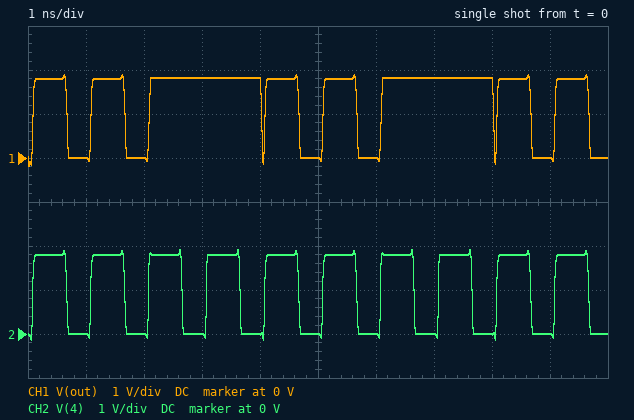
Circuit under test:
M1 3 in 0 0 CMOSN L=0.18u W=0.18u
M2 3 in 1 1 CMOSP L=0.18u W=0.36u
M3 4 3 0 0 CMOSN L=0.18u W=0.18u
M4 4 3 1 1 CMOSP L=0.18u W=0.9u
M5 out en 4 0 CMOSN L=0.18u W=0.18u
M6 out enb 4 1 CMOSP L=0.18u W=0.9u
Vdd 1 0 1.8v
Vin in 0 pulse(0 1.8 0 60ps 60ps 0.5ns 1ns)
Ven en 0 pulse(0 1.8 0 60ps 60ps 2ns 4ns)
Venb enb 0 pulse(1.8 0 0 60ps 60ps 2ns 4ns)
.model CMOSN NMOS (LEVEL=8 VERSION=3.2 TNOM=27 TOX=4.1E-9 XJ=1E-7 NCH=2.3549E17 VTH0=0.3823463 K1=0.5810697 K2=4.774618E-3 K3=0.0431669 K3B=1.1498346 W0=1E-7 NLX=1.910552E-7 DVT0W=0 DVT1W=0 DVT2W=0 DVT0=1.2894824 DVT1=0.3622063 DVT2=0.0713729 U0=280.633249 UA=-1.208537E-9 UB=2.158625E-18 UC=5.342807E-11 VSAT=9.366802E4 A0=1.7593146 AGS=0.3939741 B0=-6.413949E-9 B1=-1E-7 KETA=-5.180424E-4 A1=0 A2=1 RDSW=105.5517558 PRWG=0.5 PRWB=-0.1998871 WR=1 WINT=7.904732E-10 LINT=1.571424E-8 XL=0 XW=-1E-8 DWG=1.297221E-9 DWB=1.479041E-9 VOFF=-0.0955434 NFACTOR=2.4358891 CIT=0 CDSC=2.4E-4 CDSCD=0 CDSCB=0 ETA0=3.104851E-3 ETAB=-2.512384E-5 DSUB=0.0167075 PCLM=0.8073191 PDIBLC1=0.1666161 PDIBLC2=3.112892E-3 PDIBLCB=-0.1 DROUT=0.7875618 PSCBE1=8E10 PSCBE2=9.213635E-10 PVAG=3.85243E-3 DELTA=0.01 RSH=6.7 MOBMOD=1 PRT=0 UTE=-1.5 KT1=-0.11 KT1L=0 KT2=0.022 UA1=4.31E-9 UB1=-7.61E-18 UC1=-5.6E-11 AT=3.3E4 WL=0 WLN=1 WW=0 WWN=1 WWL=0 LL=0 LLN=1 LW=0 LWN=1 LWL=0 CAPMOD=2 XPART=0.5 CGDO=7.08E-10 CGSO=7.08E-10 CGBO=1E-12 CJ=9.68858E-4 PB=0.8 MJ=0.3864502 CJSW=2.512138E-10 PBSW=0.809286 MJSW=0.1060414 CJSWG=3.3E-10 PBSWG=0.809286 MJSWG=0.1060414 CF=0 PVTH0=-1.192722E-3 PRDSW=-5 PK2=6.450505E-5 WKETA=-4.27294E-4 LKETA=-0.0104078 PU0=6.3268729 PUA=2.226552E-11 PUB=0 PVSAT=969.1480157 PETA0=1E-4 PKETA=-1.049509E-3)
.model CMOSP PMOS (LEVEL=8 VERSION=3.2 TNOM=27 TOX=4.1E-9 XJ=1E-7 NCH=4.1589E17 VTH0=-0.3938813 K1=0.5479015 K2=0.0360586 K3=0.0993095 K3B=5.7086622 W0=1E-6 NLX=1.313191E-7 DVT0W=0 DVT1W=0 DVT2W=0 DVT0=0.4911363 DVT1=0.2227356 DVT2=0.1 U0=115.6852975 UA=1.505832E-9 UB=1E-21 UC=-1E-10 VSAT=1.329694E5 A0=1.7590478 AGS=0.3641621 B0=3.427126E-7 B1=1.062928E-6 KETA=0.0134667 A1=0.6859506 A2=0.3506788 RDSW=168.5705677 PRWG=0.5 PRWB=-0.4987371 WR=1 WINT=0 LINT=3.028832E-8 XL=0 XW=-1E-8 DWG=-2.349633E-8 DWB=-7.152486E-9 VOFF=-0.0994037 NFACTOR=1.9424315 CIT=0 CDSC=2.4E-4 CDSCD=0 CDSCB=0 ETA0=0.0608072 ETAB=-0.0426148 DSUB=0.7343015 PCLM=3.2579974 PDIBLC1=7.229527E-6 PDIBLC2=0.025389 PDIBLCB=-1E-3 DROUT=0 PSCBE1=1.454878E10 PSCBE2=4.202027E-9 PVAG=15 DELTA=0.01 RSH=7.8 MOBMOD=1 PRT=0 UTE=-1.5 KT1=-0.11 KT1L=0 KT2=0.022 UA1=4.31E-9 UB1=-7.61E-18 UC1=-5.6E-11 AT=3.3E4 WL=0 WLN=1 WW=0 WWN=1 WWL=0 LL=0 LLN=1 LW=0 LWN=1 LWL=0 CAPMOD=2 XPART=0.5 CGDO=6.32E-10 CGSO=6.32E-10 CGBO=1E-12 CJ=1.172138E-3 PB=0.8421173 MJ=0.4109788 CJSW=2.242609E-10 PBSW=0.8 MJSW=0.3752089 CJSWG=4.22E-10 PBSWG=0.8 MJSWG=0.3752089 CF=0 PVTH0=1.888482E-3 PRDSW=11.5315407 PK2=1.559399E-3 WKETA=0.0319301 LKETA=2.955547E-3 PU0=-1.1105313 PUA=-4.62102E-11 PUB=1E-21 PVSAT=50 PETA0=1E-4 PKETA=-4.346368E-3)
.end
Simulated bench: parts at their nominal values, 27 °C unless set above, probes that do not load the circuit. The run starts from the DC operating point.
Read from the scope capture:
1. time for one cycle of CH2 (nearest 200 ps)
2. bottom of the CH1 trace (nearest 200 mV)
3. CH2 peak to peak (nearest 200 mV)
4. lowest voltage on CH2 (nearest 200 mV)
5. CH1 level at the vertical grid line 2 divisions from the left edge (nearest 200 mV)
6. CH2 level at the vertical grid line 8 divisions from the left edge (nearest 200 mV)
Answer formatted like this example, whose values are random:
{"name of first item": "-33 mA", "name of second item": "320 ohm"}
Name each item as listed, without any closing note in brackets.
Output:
{"time for one cycle of CH2": "1.0 ns", "bottom of the CH1 trace": "-200 mV", "CH2 peak to peak": "2.0 V", "lowest voltage on CH2": "-200 mV", "CH1 level at the vertical grid line 2 divisions from the left edge": "0 V", "CH2 level at the vertical grid line 8 divisions from the left edge": "0 V"}
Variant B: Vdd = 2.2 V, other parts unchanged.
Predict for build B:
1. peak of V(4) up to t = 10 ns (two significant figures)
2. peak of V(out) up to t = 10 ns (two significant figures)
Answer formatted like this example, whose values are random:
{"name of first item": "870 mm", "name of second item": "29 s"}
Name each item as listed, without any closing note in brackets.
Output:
{"peak of V(4) up to t = 10 ns": "2.3 V", "peak of V(out) up to t = 10 ns": "2.4 V"}
